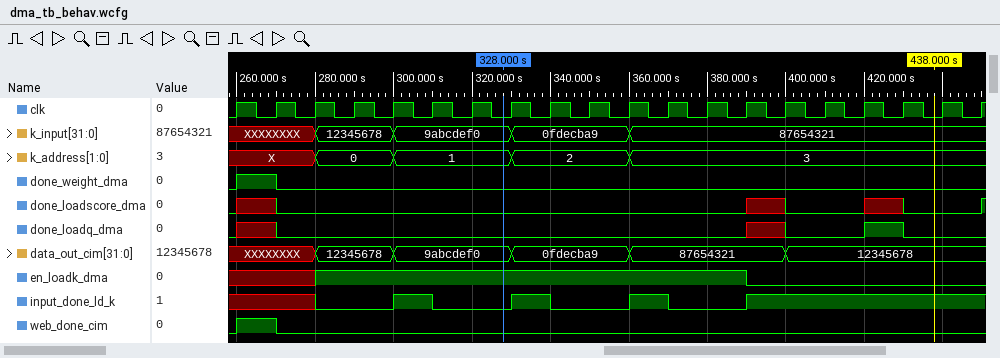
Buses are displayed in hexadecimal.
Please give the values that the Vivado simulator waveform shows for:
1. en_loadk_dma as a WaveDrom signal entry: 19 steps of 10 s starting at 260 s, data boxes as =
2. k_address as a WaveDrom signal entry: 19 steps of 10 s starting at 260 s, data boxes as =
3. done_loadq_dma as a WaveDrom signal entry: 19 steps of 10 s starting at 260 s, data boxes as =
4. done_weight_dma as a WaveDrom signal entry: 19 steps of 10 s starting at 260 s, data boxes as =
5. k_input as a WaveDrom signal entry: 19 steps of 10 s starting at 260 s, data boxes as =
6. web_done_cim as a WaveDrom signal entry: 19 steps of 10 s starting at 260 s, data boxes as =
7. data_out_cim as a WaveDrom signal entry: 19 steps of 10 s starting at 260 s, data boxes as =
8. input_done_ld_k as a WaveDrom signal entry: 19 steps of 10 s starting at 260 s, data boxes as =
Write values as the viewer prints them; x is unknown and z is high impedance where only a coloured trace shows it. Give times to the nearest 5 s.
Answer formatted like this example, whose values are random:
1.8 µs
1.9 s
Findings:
{name: 'en_loadk_dma', wave: 'x.1..........0.....'}
{name: 'k_address', wave: 'x.=.=..=..=........', data: '0 1 2 3'}
{name: 'done_loadq_dma', wave: 'x0...........x0.10.'}
{name: 'done_weight_dma', wave: '10.................'}
{name: 'k_input', wave: 'x.=.=..=..=........', data: '12345678 9abcdef0 0fdecba9 87654321'}
{name: 'web_done_cim', wave: '10.................'}
{name: 'data_out_cim', wave: 'x.=.=..=..=...=....', data: '12345678 9abcdef0 0fdecba9 87654321 12345678'}
{name: 'input_done_ld_k', wave: 'x.0.10.10.10.1.....'}
